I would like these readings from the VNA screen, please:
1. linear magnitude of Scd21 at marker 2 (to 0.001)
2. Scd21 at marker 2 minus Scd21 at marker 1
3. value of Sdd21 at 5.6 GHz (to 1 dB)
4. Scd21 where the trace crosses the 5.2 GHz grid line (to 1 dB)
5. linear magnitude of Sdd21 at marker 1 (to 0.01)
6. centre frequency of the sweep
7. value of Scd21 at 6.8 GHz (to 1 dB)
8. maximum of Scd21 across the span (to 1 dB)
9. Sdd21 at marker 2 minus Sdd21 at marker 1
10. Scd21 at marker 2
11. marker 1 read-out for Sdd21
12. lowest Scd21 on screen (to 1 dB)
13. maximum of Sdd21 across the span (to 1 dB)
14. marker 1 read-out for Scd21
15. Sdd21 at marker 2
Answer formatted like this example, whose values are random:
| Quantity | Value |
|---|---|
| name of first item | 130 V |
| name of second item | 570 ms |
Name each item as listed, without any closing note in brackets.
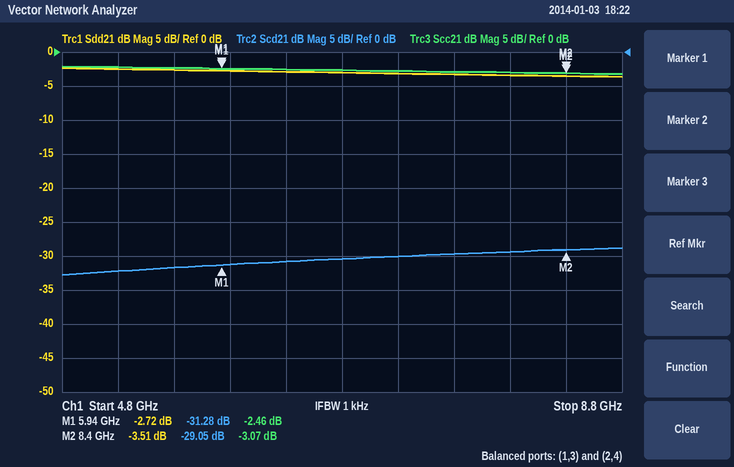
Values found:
| Quantity | Value |
|---|---|
| linear magnitude of Scd21 at marker 2 | 0.035 |
| Scd21 at marker 2 minus Scd21 at marker 1 | 2.23 dB |
| value of Sdd21 at 5.6 GHz | -3 dB |
| Scd21 where the trace crosses the 5.2 GHz grid line | -32 dB |
| linear magnitude of Sdd21 at marker 1 | 0.73 |
| centre frequency of the sweep | 6.8 GHz |
| value of Scd21 at 6.8 GHz | -30 dB |
| maximum of Scd21 across the span | -29 dB |
| Sdd21 at marker 2 minus Sdd21 at marker 1 | -0.79 dB |
| Scd21 at marker 2 | -29.05 dB |
| marker 1 read-out for Sdd21 | -2.72 dB |
| lowest Scd21 on screen | -33 dB |
| maximum of Sdd21 across the span | -2 dB |
| marker 1 read-out for Scd21 | -31.28 dB |
| Sdd21 at marker 2 | -3.51 dB |
